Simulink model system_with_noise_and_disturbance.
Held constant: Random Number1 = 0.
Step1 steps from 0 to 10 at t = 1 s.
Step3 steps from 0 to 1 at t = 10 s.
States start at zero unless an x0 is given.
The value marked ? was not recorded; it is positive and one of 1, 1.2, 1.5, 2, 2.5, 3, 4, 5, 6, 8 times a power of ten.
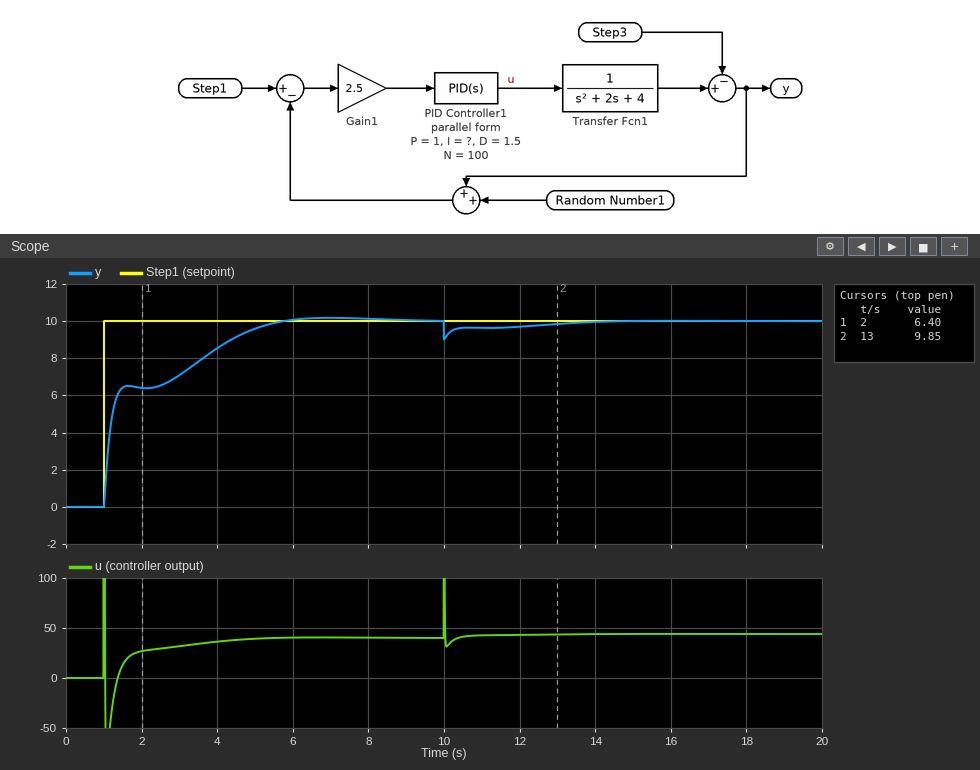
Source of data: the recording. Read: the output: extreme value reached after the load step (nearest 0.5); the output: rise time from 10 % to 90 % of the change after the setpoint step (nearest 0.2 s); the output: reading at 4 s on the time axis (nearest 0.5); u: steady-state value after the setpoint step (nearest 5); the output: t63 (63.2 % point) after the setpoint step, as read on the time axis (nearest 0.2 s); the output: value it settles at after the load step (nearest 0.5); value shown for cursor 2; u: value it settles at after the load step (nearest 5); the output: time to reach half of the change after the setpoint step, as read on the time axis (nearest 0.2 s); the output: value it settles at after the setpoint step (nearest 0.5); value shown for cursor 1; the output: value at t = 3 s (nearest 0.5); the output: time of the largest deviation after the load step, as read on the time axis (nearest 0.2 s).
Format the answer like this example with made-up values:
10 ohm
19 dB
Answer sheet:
9.0
3.4 s
8.5
40
1.4 s
10.0
9.85
45
1.2 s
10.0
6.40
7.0
10.0 s
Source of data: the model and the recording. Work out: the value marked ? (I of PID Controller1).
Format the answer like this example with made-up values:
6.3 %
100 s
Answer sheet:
1.5
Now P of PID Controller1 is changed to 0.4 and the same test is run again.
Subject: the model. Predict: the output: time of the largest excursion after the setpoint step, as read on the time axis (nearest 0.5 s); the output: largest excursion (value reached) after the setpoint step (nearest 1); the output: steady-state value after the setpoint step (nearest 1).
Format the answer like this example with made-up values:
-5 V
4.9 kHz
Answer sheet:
6.5 s
11
10
